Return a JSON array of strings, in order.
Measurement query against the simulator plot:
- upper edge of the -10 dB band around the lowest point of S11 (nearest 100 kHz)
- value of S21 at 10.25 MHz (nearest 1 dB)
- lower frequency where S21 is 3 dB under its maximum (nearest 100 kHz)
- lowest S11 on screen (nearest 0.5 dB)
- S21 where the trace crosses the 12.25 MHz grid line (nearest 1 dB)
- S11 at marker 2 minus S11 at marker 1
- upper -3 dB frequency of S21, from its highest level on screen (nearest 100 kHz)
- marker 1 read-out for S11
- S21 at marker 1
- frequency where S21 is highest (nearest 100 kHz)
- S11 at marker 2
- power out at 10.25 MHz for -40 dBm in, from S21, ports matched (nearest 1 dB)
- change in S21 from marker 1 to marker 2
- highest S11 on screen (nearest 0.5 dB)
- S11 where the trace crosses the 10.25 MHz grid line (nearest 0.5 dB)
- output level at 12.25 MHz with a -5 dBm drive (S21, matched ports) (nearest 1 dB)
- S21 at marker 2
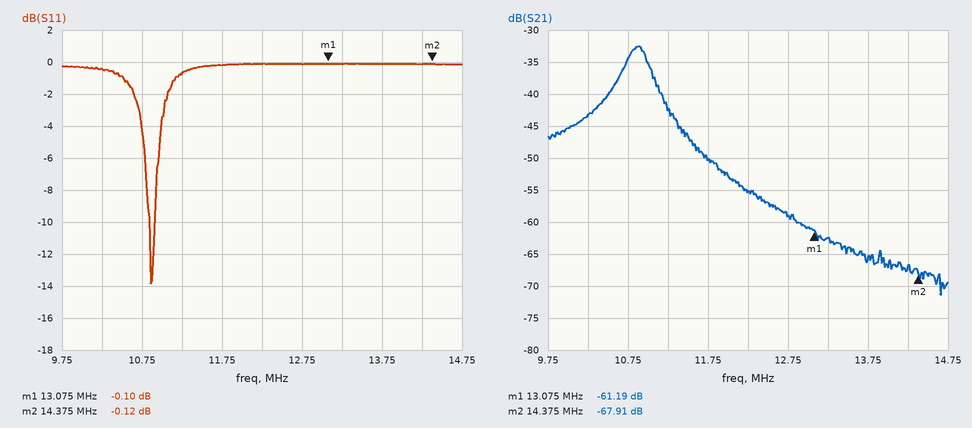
["10.9 MHz", "-43 dB", "10.7 MHz", "-14.0 dB", "-55 dB", "-0.02 dB", "11.0 MHz", "-0.10 dB", "-61.19 dB", "10.9 MHz", "-0.12 dB", "-83 dBm", "-6.72 dB", "0.0 dB", "-0.5 dB", "-60 dBm", "-67.91 dB"]
